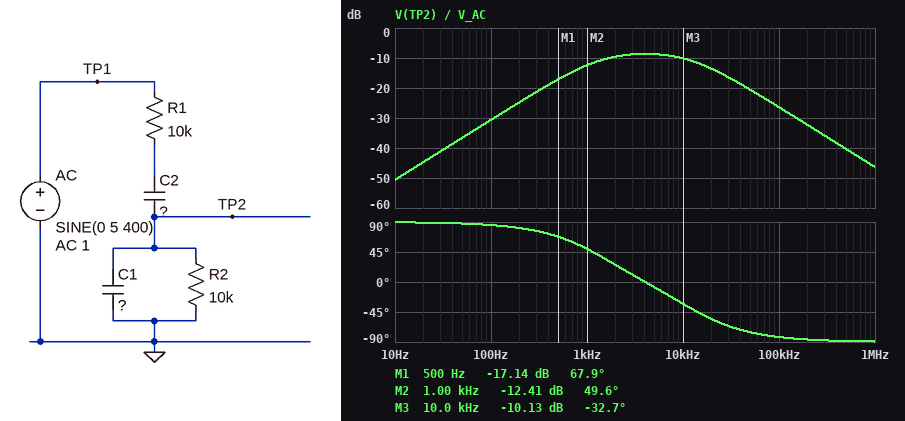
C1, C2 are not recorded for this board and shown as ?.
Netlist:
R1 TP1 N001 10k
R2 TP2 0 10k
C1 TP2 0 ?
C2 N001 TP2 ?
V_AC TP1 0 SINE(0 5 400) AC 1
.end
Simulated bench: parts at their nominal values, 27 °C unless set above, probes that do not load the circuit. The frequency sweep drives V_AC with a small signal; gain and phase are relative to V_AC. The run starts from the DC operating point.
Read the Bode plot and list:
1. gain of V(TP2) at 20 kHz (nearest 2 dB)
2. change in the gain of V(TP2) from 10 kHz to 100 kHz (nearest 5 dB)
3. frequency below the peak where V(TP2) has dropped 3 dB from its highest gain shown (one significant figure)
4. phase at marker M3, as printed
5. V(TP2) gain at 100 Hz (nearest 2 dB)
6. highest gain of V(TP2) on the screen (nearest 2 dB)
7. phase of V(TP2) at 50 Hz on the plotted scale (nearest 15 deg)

-14 dB
-15 dB
1 kHz
-32.7 deg
-30 dB
-8 dB
90 deg
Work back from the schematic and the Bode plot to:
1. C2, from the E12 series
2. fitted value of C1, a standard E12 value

4.7 nF
3.3 nF
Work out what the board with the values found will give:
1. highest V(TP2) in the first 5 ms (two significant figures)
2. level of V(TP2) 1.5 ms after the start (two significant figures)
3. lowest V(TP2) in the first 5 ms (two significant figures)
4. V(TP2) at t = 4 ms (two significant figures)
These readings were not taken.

570 mV
-540 mV
-570 mV
-540 mV
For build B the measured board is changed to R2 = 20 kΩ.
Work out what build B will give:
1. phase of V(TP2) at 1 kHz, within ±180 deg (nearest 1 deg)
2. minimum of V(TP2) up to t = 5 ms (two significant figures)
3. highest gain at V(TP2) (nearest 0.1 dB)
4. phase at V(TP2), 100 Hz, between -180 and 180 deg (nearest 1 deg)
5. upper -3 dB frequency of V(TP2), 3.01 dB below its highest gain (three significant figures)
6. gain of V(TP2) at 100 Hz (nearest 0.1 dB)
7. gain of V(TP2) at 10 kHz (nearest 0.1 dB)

34 deg
-1.1 V
-6.9 dB
83 deg
11.3 kHz
-24.6 dB
-9.3 dB
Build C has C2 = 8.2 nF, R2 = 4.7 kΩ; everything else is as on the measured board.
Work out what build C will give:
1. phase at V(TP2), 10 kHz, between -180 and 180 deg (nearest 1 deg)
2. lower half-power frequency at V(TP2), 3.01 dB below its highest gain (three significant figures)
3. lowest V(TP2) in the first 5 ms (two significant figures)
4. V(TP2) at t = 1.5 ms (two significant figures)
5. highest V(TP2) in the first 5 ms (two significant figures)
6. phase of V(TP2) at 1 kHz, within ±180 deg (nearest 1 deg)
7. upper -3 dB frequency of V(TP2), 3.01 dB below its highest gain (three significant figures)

-25 deg
1.10 kHz
-460 mV
-440 mV
460 mV
48 deg
18.1 kHz
